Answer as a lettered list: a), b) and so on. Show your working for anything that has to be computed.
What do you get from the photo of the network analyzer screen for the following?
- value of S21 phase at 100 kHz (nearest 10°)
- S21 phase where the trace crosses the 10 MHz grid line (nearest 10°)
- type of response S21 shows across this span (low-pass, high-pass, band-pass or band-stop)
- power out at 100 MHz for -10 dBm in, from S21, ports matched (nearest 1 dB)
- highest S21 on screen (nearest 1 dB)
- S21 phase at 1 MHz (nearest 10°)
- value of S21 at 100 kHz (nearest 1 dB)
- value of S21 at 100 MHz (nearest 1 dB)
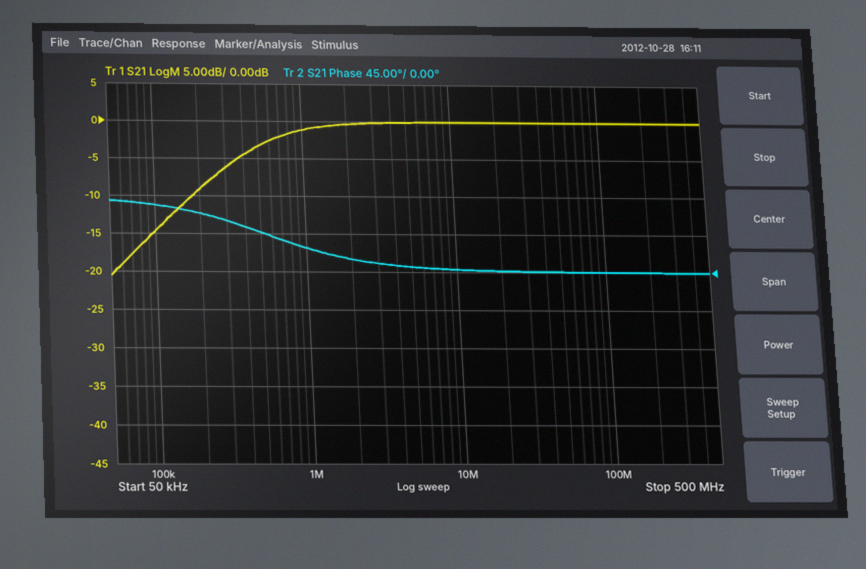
a) 80°
b) 0°
c) high-pass
d) -10 dBm + (0 dB) = -10 dBm
e) 0 dB
f) 30°
g) -15 dB
h) 0 dB
